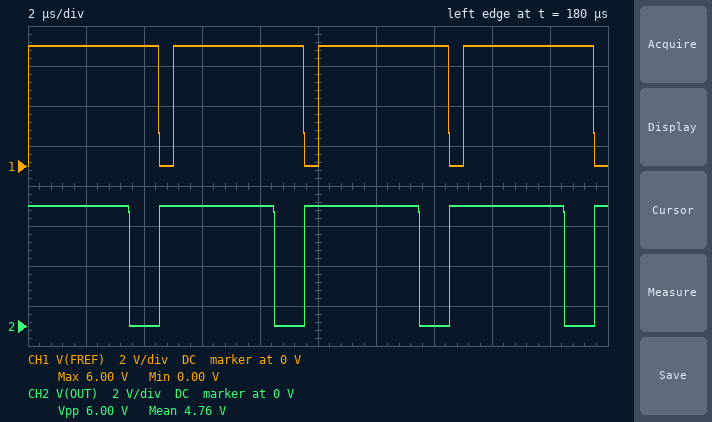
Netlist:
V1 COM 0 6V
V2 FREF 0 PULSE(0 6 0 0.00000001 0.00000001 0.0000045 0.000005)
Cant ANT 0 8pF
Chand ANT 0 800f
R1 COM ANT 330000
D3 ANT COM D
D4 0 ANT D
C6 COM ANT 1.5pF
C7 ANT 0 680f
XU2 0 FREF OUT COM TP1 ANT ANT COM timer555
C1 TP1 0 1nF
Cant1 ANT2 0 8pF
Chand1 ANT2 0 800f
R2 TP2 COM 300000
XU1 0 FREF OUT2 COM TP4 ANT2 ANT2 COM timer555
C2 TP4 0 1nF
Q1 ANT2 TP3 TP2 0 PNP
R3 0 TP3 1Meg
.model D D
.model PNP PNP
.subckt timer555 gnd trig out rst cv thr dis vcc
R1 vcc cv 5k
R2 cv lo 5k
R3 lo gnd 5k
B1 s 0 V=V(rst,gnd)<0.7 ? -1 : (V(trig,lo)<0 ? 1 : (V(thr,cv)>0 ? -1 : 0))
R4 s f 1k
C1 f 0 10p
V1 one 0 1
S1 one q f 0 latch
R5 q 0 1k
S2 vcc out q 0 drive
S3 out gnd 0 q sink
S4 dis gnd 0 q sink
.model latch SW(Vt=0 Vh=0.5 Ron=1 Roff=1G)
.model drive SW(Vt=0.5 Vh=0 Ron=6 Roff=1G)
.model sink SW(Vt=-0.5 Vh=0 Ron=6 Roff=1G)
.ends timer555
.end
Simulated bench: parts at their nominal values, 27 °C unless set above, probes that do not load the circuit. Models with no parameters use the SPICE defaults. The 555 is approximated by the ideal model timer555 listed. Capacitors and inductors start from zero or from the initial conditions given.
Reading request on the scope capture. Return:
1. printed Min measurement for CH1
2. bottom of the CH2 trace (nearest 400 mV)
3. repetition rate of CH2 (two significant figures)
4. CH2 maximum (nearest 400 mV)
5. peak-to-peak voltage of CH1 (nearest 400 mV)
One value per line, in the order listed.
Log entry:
0.00 V
0 V
200 kHz
6.0 V
6.0 V
